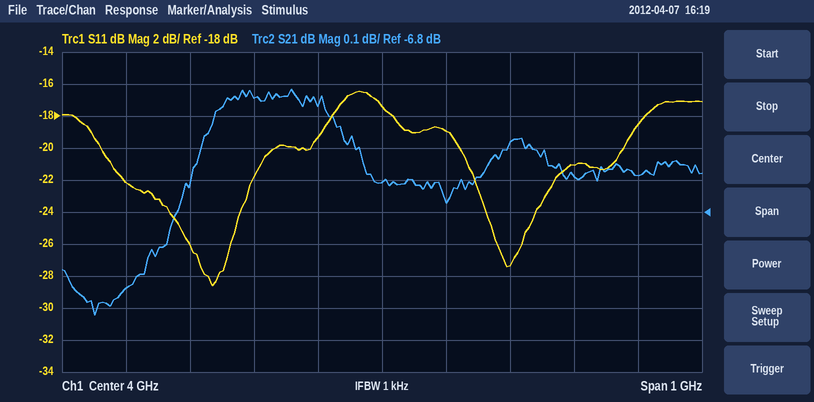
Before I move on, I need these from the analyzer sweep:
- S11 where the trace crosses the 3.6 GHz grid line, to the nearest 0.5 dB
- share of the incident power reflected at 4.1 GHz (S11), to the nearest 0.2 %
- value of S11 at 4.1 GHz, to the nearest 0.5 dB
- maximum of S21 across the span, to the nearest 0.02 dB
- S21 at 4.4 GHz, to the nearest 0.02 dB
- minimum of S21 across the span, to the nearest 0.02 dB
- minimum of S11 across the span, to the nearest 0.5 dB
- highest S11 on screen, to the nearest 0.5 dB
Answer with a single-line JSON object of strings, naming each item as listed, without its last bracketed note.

{"S11 where the trace crosses the 3.6 GHz grid line, to the nearest 0.5 dB": "-22.0 dB", "share of the incident power reflected at 4.1 GHz (S11), to the nearest 0.2 %": "1.2 %", "value of S11 at 4.1 GHz, to the nearest 0.5 dB": "-19.0 dB", "maximum of S21 across the span, to the nearest 0.02 dB": "-6.42 dB", "S21 at 4.4 GHz, to the nearest 0.02 dB": "-6.68 dB", "minimum of S21 across the span, to the nearest 0.02 dB": "-7.12 dB", "minimum of S11 across the span, to the nearest 0.5 dB": "-28.5 dB", "highest S11 on screen, to the nearest 0.5 dB": "-16.5 dB"}
